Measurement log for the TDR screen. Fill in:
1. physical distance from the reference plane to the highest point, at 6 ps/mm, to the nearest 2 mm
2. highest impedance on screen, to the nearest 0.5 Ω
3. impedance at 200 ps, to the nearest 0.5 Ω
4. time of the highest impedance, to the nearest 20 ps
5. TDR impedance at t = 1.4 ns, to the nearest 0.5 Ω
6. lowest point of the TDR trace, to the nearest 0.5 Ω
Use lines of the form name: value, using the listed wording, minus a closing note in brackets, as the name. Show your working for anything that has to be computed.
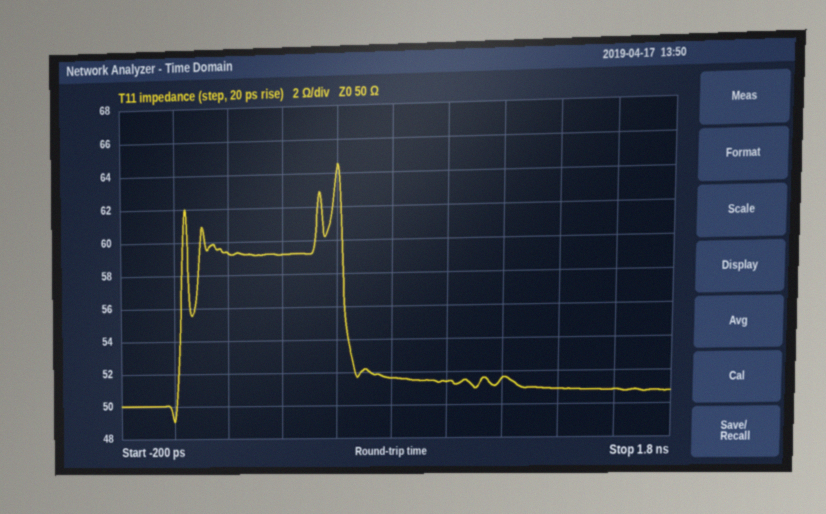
physical distance from the reference plane to the highest point, at 6 ps/mm, to the nearest 2 mm: 600 ps / 2 / 6 ps/mm ≈ 50 mm
highest impedance on screen, to the nearest 0.5 Ω: 64.5 Ω
impedance at 200 ps, to the nearest 0.5 Ω: 59.5 Ω
time of the highest impedance, to the nearest 20 ps: 600 ps
TDR impedance at t = 1.4 ns, to the nearest 0.5 Ω: 51.0 Ω
lowest point of the TDR trace, to the nearest 0.5 Ω: 49.0 Ω
